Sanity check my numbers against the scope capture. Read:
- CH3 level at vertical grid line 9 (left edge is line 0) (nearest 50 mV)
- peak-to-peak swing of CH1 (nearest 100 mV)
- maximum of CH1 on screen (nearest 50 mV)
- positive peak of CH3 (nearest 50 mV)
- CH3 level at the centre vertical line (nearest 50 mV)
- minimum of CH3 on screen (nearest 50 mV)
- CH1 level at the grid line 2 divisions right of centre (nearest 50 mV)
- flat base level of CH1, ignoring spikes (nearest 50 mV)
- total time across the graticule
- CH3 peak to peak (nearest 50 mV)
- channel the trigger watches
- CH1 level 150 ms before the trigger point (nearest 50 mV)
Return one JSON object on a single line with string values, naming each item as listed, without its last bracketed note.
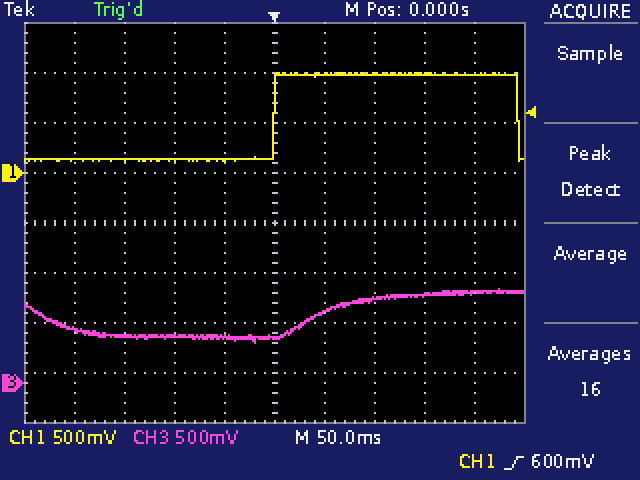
{"CH3 level at vertical grid line 9 (left edge is line 0)": "900 mV", "peak-to-peak swing of CH1": "900 mV", "maximum of CH1 on screen": "1.00 V", "positive peak of CH3": "950 mV", "CH3 level at the centre vertical line": "450 mV", "minimum of CH3 on screen": "400 mV", "CH1 level at the grid line 2 divisions right of centre": "1.00 V", "flat base level of CH1, ignoring spikes": "150 mV", "total time across the graticule": "500 ms", "CH3 peak to peak": "550 mV", "channel the trigger watches": "CH1", "CH1 level 150 ms before the trigger point": "150 mV"}
